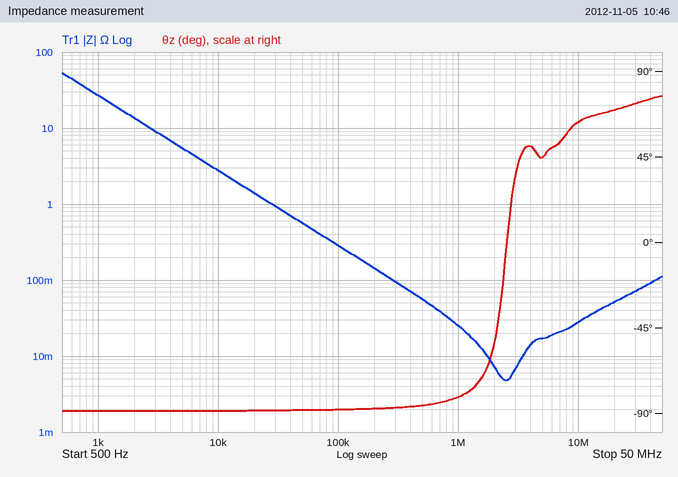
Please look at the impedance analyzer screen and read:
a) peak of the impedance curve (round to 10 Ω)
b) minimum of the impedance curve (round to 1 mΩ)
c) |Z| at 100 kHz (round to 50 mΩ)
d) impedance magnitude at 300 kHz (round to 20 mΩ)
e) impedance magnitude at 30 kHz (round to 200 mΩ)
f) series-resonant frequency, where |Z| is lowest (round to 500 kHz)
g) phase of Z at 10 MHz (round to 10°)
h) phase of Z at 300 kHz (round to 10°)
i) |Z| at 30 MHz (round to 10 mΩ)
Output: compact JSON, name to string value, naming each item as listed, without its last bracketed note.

{"peak of the impedance curve": "50 Ω", "minimum of the impedance curve": "5 mΩ", "|Z| at 100 kHz": "300 mΩ", "impedance magnitude at 300 kHz": "100 mΩ", "impedance magnitude at 30 kHz": "1.0 Ω", "series-resonant frequency, where |Z| is lowest": "2.5 MHz", "phase of Z at 10 MHz": "60°", "phase of Z at 300 kHz": "-90°", "|Z| at 30 MHz": "70 mΩ"}
